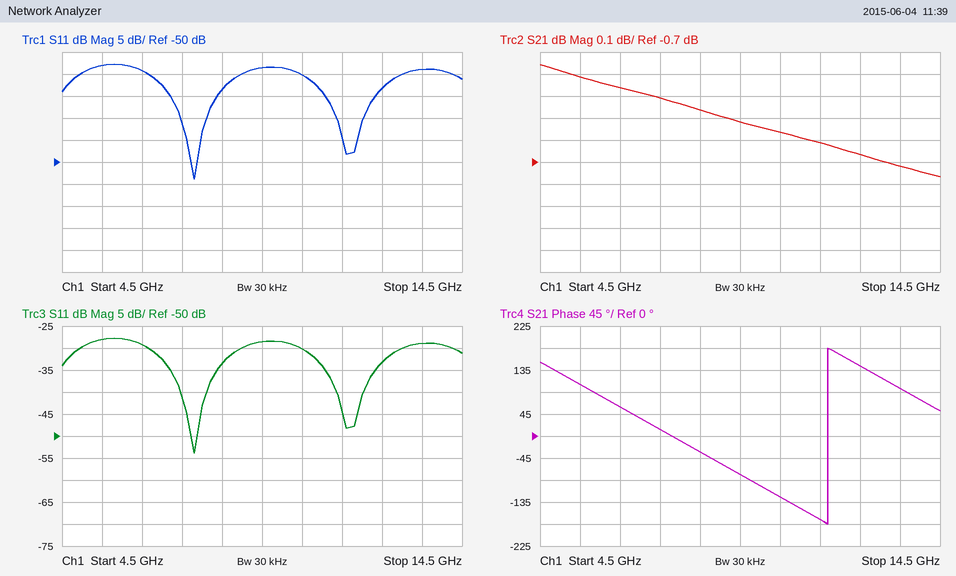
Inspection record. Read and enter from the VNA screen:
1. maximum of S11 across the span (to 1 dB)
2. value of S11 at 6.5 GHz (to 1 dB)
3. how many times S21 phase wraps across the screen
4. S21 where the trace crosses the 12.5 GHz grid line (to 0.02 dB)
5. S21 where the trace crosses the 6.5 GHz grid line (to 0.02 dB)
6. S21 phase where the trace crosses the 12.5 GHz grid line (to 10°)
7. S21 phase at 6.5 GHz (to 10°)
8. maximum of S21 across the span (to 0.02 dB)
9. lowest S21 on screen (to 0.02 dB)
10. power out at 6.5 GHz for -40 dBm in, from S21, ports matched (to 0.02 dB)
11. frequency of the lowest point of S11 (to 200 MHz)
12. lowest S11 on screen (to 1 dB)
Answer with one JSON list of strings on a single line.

["-28 dB", "-29 dB", "1", "-0.66 dB", "-0.36 dB", "140°", "60°", "-0.26 dB", "-0.76 dB", "-40.36 dBm", "7.8 GHz", "-54 dB"]
